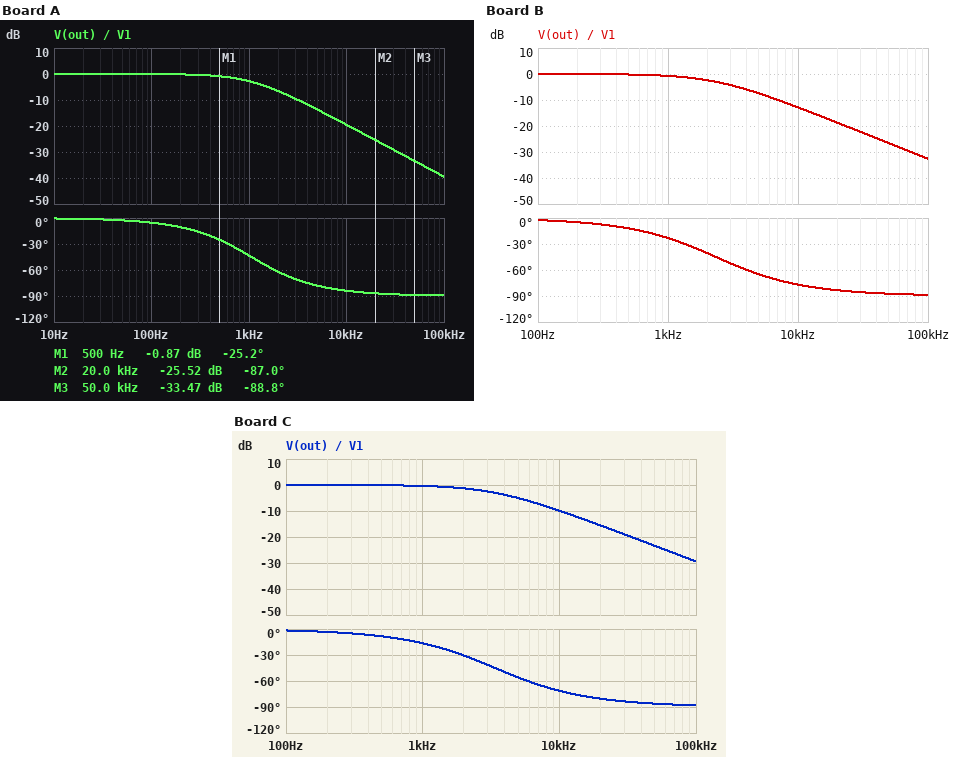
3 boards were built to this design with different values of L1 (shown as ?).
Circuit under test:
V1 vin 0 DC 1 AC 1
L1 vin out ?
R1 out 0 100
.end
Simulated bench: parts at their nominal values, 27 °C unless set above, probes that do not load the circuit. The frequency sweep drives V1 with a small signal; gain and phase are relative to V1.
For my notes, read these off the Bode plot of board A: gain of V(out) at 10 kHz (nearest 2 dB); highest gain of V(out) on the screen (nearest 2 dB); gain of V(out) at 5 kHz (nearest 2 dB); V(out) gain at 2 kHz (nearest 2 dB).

-20 dB
0 dB
-14 dB
-6 dB
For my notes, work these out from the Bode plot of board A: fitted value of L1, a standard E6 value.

15 mH
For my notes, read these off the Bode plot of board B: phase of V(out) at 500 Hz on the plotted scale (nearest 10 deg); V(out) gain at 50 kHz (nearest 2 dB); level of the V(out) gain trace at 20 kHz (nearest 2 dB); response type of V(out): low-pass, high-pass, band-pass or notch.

-10 deg
-26 dB
-18 dB
low-pass
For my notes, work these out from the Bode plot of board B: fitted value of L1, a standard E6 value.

6.8 mH
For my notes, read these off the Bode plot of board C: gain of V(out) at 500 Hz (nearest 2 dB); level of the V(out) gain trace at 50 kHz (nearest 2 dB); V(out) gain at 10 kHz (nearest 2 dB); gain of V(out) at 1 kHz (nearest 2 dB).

0 dB
-24 dB
-10 dB
0 dB
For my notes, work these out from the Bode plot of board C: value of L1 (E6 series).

4.7 mH
